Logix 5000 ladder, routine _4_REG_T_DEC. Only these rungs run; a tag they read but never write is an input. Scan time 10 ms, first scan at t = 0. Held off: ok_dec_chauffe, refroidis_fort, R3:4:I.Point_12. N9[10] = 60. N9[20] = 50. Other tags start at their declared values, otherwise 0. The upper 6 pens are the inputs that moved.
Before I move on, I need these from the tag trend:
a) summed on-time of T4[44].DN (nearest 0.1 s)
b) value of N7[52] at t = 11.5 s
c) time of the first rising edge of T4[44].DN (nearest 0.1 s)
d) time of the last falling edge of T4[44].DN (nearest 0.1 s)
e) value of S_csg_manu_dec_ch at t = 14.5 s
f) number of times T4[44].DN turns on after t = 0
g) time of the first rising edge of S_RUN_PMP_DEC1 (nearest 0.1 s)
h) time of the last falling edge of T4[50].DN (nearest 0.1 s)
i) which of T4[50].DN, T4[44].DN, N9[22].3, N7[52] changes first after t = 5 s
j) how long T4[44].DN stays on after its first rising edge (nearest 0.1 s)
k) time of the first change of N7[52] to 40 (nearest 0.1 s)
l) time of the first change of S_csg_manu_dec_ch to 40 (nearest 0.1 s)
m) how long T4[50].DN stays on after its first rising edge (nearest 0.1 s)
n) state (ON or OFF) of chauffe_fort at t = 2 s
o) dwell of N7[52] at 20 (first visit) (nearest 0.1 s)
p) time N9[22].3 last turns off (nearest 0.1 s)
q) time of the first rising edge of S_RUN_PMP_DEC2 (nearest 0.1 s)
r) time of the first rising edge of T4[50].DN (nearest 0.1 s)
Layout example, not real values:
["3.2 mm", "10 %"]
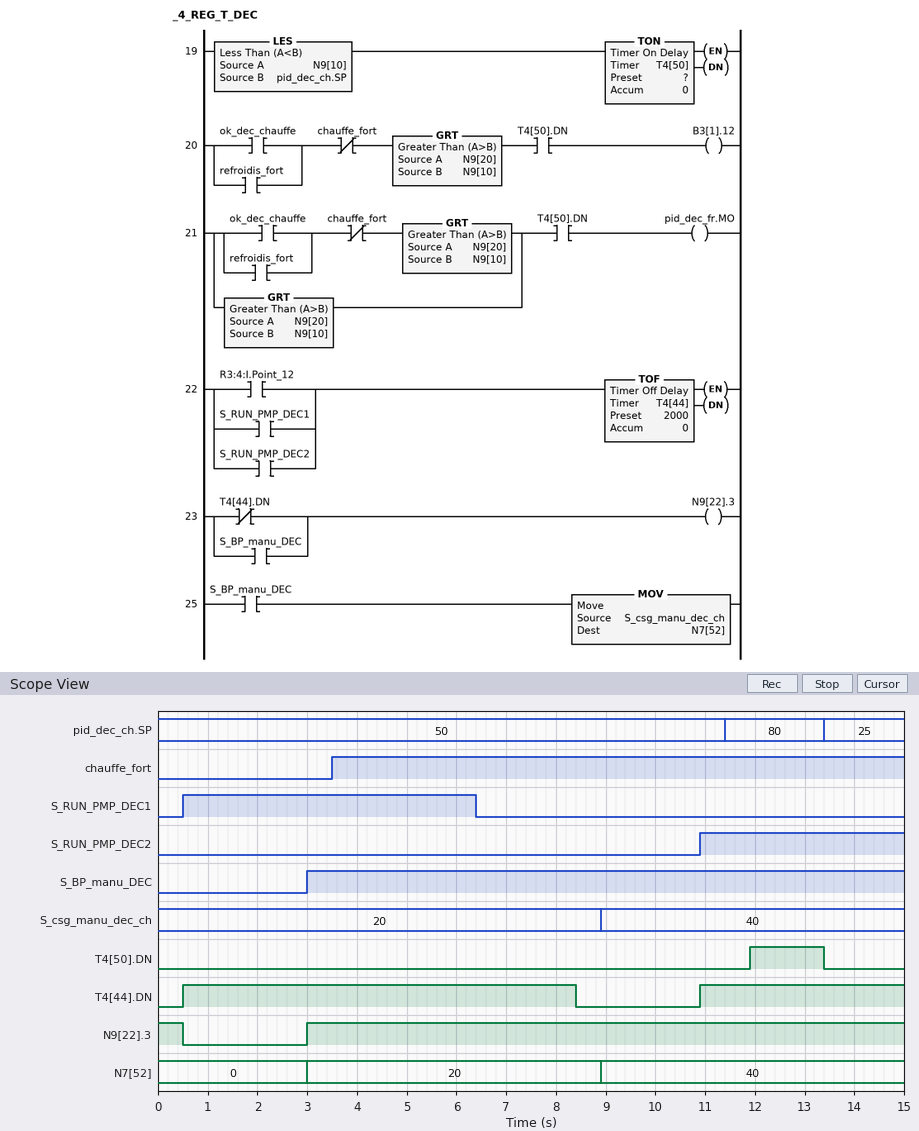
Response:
["12.0 s", "40", "0.5 s", "8.4 s", "40", "2", "0.5 s", "13.4 s", "T4[44].DN", "7.9 s", "8.9 s", "8.9 s", "1.5 s", "OFF", "5.9 s", "0.5 s", "10.9 s", "11.9 s"]
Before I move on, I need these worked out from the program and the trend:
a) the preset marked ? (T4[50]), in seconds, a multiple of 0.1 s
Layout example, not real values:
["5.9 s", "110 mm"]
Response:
["0.5 s"]
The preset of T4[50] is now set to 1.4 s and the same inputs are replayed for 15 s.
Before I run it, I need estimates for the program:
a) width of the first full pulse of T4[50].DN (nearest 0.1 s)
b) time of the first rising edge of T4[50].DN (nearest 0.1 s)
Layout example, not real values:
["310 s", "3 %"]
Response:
["0.6 s", "12.8 s"]
